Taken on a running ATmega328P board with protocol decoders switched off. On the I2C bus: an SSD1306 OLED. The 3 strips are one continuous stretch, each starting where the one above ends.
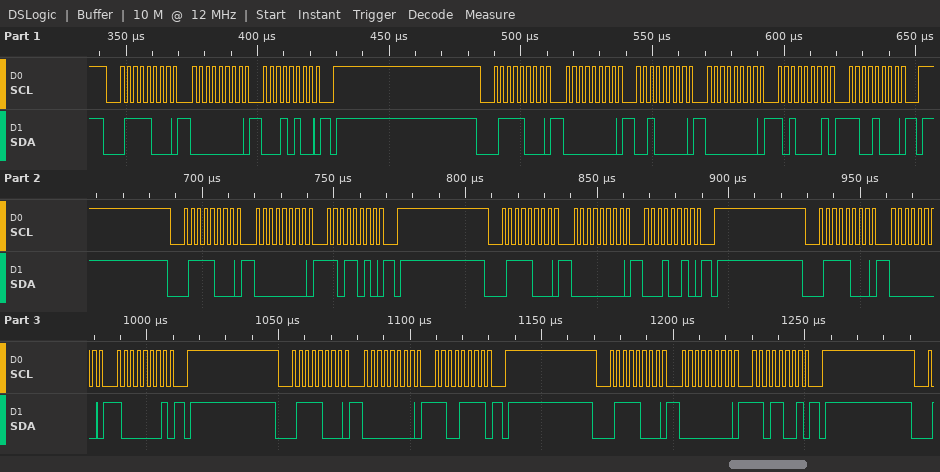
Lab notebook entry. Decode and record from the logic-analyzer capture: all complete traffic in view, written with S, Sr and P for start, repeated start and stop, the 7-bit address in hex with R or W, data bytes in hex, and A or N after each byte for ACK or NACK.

S 3CW A 00 A 14 A P S 3CW A 00 A 20 A 00 A A1 A C8 A P S 3CW A 00 A DA A P S 3CW A 00 A 12 A P S 3CW A 00 A 81 A P S 3CW A 00 A CF A P S 3CW A 00 A D9 A P
